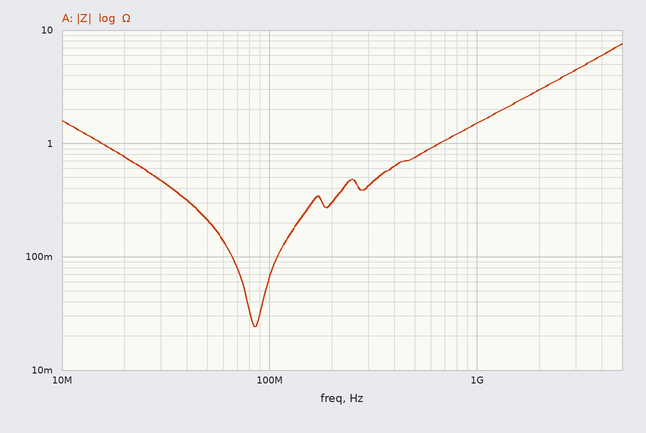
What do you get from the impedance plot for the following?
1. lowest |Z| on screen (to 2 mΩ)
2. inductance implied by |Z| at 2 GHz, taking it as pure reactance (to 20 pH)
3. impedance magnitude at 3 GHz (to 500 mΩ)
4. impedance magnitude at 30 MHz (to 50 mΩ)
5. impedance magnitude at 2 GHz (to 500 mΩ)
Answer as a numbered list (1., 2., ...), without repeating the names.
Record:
1. 24 mΩ
2. 240 pH
3. 4.5 Ω
4. 450 mΩ
5. 3.0 Ω
